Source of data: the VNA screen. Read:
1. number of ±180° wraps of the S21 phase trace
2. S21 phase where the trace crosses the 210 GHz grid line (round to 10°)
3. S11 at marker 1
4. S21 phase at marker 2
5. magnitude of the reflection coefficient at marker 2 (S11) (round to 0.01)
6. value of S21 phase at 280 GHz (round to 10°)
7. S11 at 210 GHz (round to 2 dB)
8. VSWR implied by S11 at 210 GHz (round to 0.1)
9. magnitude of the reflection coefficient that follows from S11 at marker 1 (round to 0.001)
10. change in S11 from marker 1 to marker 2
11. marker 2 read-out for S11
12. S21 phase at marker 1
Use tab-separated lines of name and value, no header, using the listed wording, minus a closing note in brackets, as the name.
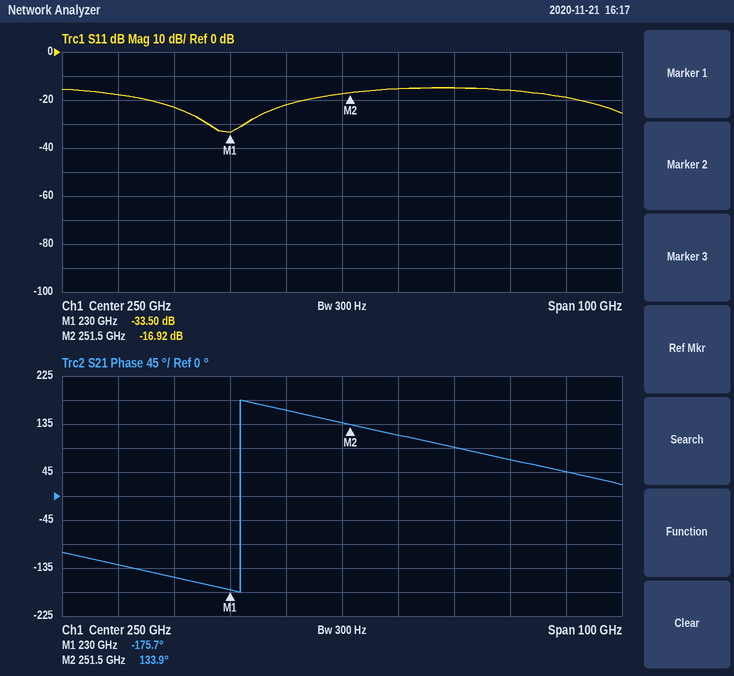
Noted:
number of ±180° wraps of the S21 phase trace	1
S21 phase where the trace crosses the 210 GHz grid line	-130°
S11 at marker 1	-33.50 dB
S21 phase at marker 2	133.9°
magnitude of the reflection coefficient at marker 2 (S11)	0.14
value of S21 phase at 280 GHz	70°
S11 at 210 GHz	-18 dB
VSWR implied by S11 at 210 GHz	1.3
magnitude of the reflection coefficient that follows from S11 at marker 1	0.021
change in S11 from marker 1 to marker 2	16.58 dB
marker 2 read-out for S11	-16.92 dB
S21 phase at marker 1	-175.7°
